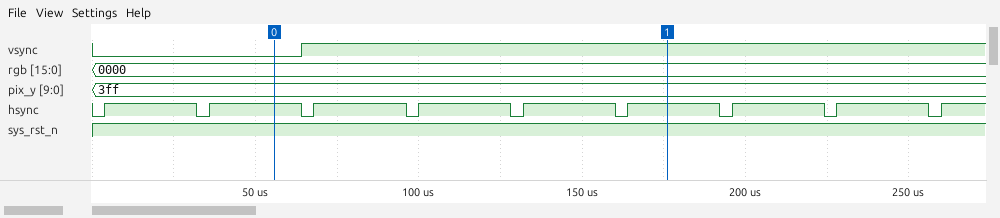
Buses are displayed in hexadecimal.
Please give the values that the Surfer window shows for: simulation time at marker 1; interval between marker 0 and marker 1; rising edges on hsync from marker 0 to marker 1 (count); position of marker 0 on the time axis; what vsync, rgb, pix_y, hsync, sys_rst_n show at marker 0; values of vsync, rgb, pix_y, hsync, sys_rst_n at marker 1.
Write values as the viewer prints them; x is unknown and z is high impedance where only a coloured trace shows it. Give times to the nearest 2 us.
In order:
176 us
120 us
4
56 us
vsync=0, rgb=0000, pix_y=3ff, hsync=1, sys_rst_n=1
vsync=1, rgb=0000, pix_y=3ff, hsync=1, sys_rst_n=1
